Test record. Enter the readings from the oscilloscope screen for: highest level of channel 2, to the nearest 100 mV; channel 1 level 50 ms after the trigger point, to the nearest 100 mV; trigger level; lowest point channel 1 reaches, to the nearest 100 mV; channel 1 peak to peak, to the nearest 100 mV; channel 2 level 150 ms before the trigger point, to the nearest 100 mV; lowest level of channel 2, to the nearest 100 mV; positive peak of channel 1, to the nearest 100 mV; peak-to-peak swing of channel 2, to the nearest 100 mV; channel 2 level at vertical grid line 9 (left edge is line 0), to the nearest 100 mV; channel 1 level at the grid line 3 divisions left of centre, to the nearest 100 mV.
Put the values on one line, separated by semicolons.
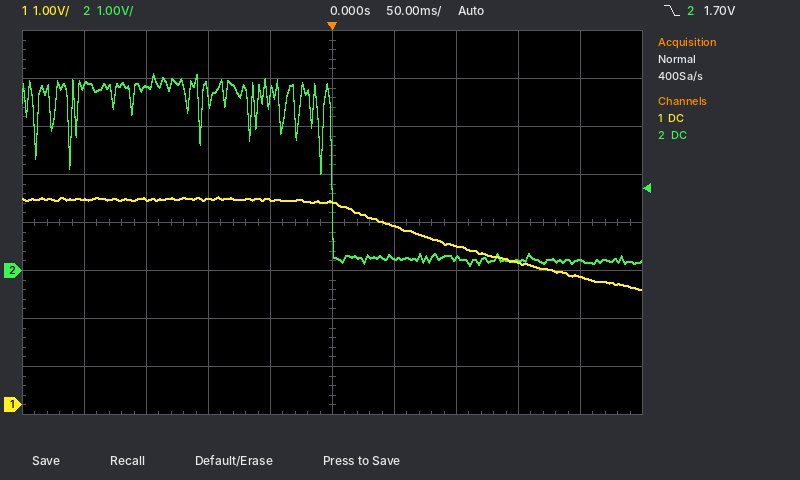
4.1 V; 3.7 V; 1.70 V; 2.4 V; 1.9 V; 3.8 V; 100 mV; 4.3 V; 4.0 V; 200 mV; 4.3 V
